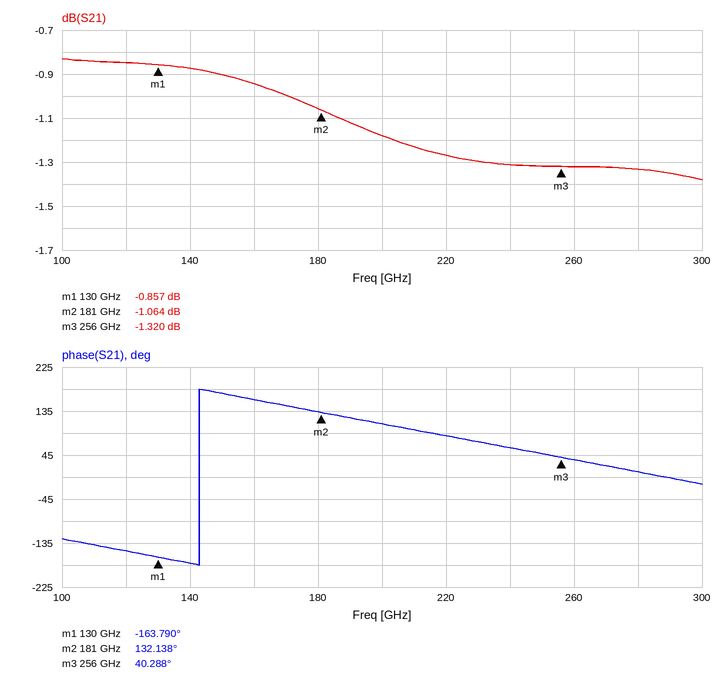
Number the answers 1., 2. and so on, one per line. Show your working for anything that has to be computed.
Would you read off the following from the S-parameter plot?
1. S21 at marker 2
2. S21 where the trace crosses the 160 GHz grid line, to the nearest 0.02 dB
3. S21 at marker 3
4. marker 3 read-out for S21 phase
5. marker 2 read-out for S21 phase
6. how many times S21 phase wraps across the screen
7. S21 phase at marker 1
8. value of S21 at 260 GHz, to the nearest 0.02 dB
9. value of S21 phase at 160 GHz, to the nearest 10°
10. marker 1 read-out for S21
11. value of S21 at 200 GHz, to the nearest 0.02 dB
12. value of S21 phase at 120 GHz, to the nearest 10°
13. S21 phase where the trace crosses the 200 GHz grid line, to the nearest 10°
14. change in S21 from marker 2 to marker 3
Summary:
1. -1.064 dB
2. -0.94 dB
3. -1.320 dB
4. 40.288°
5. 132.138°
6. 1
7. -163.790°
8. -1.32 dB
9. 160°
10. -0.857 dB
11. -1.18 dB
12. -150°
13. 110°
14. -1.32 − (-1.064) = -0.256 dB
